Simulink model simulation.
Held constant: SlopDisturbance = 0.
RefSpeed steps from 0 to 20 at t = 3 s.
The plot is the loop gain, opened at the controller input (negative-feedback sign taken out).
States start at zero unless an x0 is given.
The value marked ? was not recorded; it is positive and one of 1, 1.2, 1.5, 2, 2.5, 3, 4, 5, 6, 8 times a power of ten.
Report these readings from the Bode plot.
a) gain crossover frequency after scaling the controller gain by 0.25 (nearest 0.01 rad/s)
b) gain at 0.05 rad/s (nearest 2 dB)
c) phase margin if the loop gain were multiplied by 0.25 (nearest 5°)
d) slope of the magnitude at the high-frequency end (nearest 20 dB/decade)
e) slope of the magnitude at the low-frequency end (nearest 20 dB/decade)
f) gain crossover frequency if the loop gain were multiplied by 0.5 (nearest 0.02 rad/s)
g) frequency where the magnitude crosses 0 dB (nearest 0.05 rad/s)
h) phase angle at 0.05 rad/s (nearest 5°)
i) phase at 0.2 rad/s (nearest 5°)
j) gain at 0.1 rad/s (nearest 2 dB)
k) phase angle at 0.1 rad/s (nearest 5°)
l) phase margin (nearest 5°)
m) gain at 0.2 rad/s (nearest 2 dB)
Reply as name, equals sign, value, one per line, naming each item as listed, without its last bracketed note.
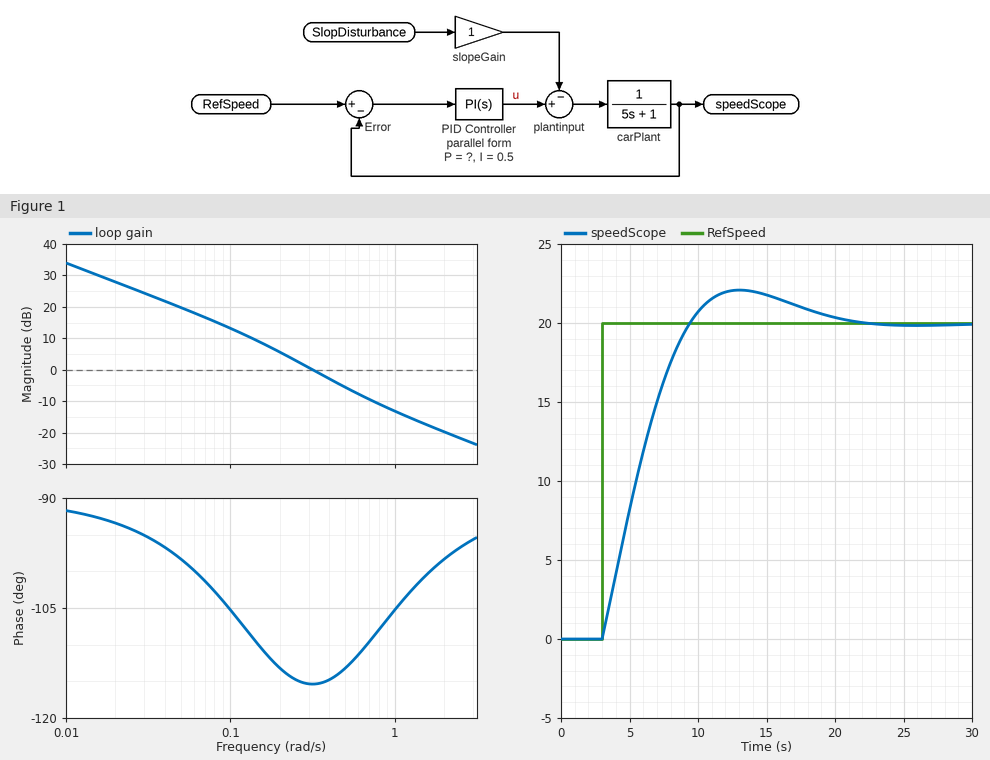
gain crossover frequency after scaling the controller gain by 0.25 = 0.11 rad/s
gain at 0.05 rad/s = 20 dB
phase margin if the loop gain were multiplied by 0.25 = 75°
slope of the magnitude at the high-frequency end = -20 dB/decade
slope of the magnitude at the low-frequency end = -20 dB/decade
gain crossover frequency if the loop gain were multiplied by 0.5 = 0.20 rad/s
frequency where the magnitude crosses 0 dB = 0.30 rad/s
phase angle at 0.05 rad/s = -100°
phase at 0.2 rad/s = -115°
gain at 0.1 rad/s = 14 dB
phase angle at 0.1 rad/s = -105°
phase margin = 65°
gain at 0.2 rad/s = 6 dB
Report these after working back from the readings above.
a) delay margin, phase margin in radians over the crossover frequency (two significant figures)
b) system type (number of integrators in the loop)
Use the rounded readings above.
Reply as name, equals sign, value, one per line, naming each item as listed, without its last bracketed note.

delay margin, phase margin in radians over the crossover frequency = 3.8 s
system type = 1
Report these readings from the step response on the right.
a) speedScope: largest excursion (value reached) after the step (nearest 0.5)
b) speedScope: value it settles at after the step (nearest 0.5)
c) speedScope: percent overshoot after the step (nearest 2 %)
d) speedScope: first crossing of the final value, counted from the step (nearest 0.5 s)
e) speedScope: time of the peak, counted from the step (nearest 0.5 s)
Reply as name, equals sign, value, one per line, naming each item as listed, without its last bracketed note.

speedScope: largest excursion (value reached) after the step = 22.0
speedScope: value it settles at after the step = 20.0
speedScope: percent overshoot after the step = 10 %
speedScope: first crossing of the final value, counted from the step = 6.5 s
speedScope: time of the peak, counted from the step = 10.0 s
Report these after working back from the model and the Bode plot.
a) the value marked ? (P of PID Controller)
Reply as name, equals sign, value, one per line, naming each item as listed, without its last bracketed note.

the value marked ? = 1
